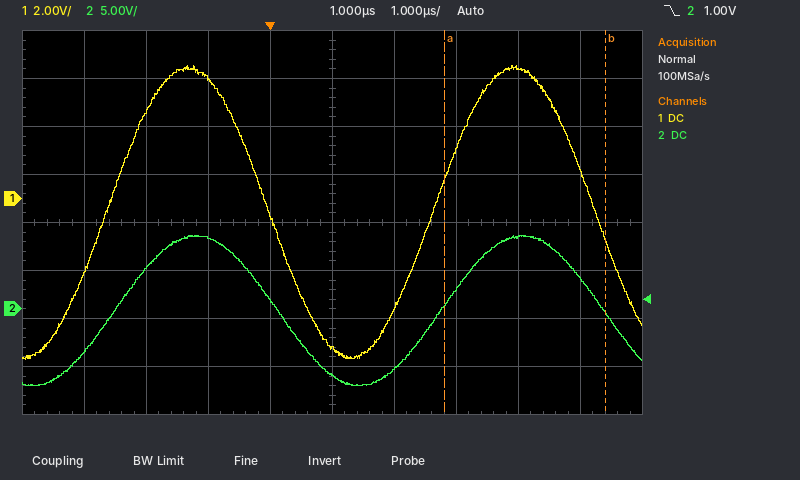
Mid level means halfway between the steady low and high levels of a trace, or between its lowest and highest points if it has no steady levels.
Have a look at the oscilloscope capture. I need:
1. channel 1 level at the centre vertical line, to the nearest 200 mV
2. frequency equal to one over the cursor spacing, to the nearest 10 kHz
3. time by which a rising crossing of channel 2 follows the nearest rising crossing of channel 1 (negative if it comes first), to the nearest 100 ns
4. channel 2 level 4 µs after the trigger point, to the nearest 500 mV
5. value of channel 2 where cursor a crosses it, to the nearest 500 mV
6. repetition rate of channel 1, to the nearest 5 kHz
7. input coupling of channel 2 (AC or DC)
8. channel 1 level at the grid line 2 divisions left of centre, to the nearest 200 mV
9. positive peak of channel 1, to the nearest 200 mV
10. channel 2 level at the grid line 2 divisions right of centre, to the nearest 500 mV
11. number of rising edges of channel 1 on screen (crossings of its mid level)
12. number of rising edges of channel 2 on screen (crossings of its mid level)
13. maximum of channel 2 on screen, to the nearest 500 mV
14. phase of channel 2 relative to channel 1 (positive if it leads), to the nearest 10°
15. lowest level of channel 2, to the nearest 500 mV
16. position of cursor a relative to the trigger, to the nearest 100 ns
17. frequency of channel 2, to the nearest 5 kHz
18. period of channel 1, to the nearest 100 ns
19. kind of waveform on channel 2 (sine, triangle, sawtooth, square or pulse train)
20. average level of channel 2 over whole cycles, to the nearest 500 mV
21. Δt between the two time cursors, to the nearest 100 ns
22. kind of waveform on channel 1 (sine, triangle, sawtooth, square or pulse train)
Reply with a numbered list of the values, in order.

1. -6.2 V
2. 380 kHz
3. +100 ns
4. 7.5 V
5. 500 mV
6. 190 kHz
7. DC
8. 5.0 V
9. 5.6 V
10. 2.0 V
11. 2
12. 2
13. 7.5 V
14. -10°
15. -8.0 V
16. +2.8 µs
17. 190 kHz
18. 5.3 µs
19. sine
20. 0.0 V
21. 2.6 µs
22. sine
